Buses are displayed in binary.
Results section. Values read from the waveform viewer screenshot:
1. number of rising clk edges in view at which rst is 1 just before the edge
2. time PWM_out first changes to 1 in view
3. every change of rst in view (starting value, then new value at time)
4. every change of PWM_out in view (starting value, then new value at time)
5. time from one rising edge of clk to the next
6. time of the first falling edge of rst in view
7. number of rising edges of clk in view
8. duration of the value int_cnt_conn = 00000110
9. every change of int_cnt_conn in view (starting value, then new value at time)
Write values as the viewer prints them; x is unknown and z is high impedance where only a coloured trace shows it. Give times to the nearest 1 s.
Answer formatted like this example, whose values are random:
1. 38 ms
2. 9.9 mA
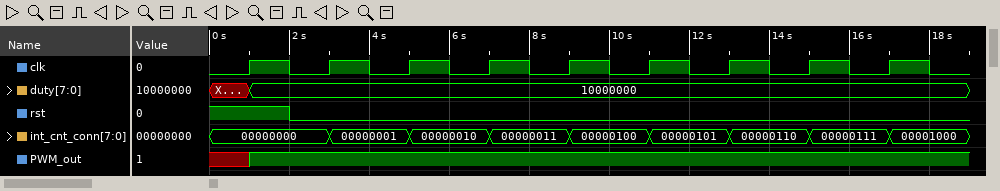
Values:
1. 1
2. 1 s
3. 1, 0 at 2 s
4. x, 1 at 1 s
5. 2 s
6. 2 s
7. 9
8. 2 s
9. 00000000, 00000001 at 3 s, 00000010 at 5 s, 00000011 at 7 s, 00000100 at 9 s, 00000101 at 11 s, 00000110 at 13 s, 00000111 at 15 s, 00001000 at 17 s
